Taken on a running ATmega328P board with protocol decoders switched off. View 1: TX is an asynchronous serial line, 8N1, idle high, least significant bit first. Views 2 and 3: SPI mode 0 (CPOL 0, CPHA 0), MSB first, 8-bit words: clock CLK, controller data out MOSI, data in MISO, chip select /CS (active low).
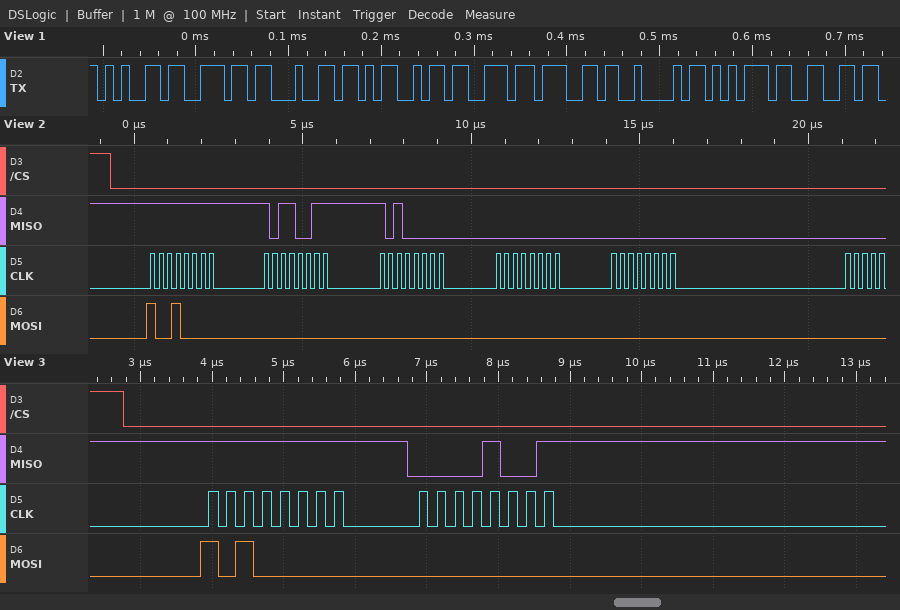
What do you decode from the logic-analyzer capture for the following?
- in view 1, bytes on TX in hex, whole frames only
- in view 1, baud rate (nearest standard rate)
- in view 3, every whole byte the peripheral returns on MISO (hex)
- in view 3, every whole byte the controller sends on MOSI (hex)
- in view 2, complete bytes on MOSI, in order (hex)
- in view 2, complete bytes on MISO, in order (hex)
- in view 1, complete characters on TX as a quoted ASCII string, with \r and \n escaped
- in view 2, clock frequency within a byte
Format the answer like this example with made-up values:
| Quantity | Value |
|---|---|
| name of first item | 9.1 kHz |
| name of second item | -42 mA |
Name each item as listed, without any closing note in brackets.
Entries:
| Quantity | Value |
|---|---|
| in view 1, bytes on TX in hex, whole frames only | 0x65 0x6E 0x64 0x4D 0x73 0x67 0x42 0x75 0x66 |
| in view 1, baud rate | 115200 baud |
| in view 3, every whole byte the peripheral returns on MISO | FF 09 |
| in view 3, every whole byte the controller sends on MOSI | A0 00 |
| in view 2, complete bytes on MOSI, in order | 0x90 0x00 0x00 0x00 0x00 |
| in view 2, complete bytes on MISO, in order | 0xFF 0xB3 0xA0 0x00 0x00 |
| in view 1, complete characters on TX as a quoted ASCII string, with \r and \n escaped | "endMsgBuf" |
| in view 2, clock frequency within a byte | 4 MHz |
